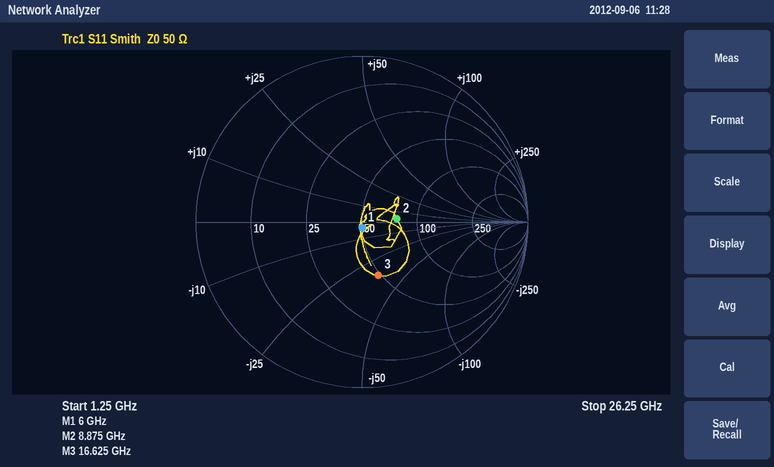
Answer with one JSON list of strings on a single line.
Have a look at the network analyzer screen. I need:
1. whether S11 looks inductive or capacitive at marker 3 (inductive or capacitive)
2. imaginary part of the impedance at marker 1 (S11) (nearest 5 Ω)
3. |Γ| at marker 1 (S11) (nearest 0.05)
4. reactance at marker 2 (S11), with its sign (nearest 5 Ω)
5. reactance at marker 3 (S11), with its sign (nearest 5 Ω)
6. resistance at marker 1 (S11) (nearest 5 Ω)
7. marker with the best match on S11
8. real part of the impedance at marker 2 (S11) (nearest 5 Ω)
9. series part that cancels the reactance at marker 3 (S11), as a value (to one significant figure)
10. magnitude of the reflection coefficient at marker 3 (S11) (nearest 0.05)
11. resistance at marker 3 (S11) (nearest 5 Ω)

["capacitive", "-5 Ω", "0.05", "+5 Ω", "-35 Ω", "50 Ω", "marker 1", "75 Ω", "300 pH", "0.35", "50 Ω"]
